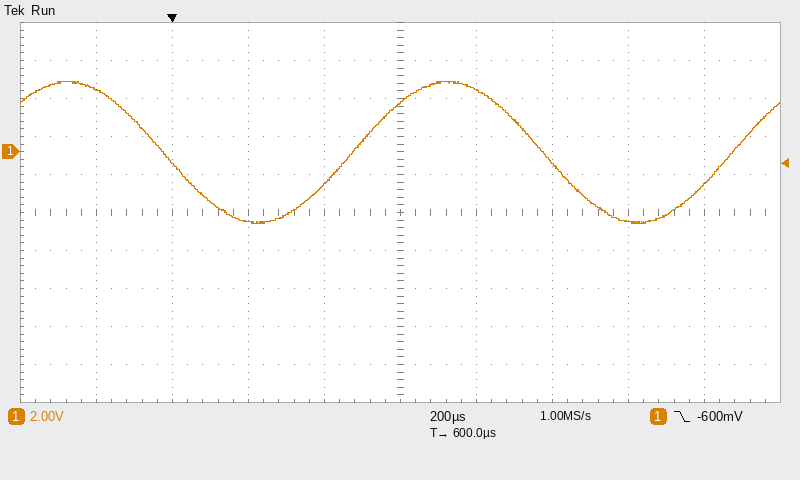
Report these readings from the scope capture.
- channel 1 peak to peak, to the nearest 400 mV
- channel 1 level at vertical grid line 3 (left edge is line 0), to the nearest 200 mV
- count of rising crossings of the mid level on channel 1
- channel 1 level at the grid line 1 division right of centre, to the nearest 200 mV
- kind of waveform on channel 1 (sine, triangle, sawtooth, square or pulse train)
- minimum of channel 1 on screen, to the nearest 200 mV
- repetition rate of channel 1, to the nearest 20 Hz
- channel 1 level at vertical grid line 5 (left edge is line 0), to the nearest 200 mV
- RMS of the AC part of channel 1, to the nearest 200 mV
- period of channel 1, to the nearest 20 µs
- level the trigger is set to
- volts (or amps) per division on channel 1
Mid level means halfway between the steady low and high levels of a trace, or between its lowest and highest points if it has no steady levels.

7.6 V
-3.6 V
2
3.2 V
sine
-3.8 V
1.00 kHz
2.6 V
2.6 V
1.00 ms
-600 mV
2 V
